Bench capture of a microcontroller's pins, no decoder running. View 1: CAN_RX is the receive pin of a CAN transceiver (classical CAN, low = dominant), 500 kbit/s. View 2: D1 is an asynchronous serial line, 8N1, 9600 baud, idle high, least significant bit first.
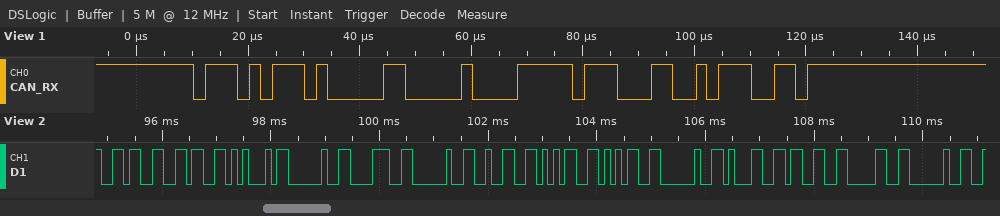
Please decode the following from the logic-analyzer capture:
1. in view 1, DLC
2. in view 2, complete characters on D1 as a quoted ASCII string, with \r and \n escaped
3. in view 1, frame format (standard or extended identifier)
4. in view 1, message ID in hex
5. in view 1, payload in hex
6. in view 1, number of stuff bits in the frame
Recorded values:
2
"66E 8 255 130 "
standard
0x75D
00 FF
3
